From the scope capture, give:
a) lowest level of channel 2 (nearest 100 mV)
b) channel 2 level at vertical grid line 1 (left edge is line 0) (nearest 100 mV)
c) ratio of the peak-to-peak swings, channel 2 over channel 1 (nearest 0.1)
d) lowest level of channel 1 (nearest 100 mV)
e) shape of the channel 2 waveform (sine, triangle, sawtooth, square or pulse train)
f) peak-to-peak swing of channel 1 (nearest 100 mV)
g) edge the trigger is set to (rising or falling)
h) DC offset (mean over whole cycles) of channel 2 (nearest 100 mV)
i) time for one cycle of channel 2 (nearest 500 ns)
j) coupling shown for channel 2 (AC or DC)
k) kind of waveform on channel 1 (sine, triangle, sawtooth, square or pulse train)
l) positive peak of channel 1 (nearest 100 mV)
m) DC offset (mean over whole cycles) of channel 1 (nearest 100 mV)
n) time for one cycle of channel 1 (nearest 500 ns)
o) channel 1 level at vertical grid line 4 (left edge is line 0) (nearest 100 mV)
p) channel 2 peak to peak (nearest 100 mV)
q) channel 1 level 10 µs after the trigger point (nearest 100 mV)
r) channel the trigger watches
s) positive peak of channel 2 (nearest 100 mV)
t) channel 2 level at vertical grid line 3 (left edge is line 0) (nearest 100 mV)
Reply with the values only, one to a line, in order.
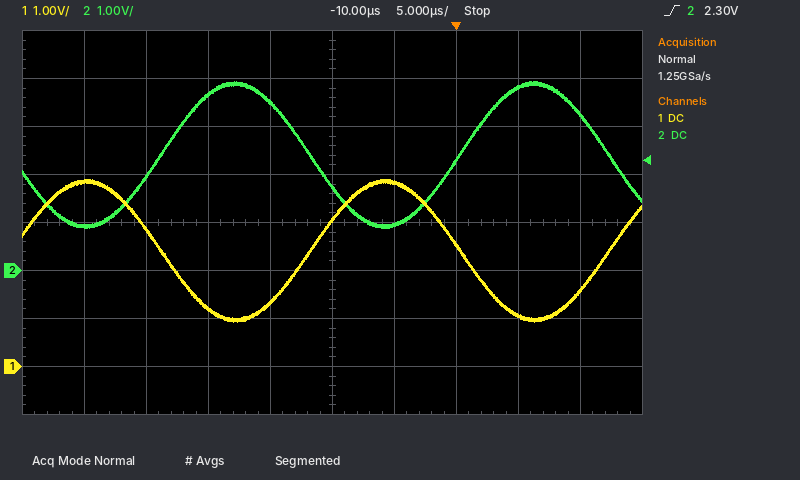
900 mV
900 mV
1.0
900 mV
sine
3.0 V
rising
2.4 V
24.0 µs
DC
sine
3.9 V
2.4 V
24.0 µs
1.3 V
3.0 V
1.6 V
channel 2
3.9 V
3.7 V
